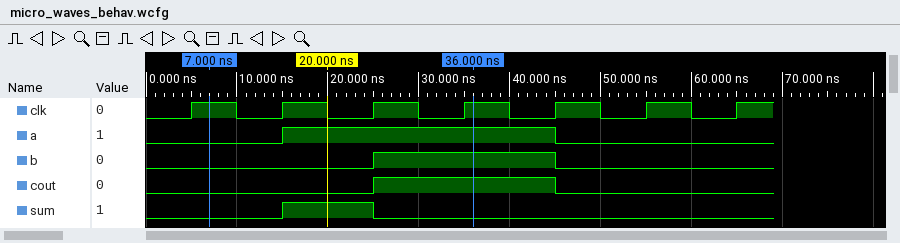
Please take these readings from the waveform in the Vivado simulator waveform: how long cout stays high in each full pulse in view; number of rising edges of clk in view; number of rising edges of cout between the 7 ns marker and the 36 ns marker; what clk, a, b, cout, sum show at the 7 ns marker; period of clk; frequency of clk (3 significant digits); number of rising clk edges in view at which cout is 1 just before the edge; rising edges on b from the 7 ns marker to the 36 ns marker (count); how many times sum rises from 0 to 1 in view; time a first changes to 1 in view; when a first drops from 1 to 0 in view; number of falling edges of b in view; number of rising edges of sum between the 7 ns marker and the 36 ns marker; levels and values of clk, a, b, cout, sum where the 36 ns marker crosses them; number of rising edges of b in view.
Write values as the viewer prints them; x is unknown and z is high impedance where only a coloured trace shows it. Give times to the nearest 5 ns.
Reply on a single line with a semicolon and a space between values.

20 ns; 7; 1; clk=1, a=0, b=0, cout=0, sum=0; 10 ns; 100 MHz; 2; 1; 1; 15 ns; 45 ns; 1; 1; clk=1, a=1, b=1, cout=1, sum=0; 1
